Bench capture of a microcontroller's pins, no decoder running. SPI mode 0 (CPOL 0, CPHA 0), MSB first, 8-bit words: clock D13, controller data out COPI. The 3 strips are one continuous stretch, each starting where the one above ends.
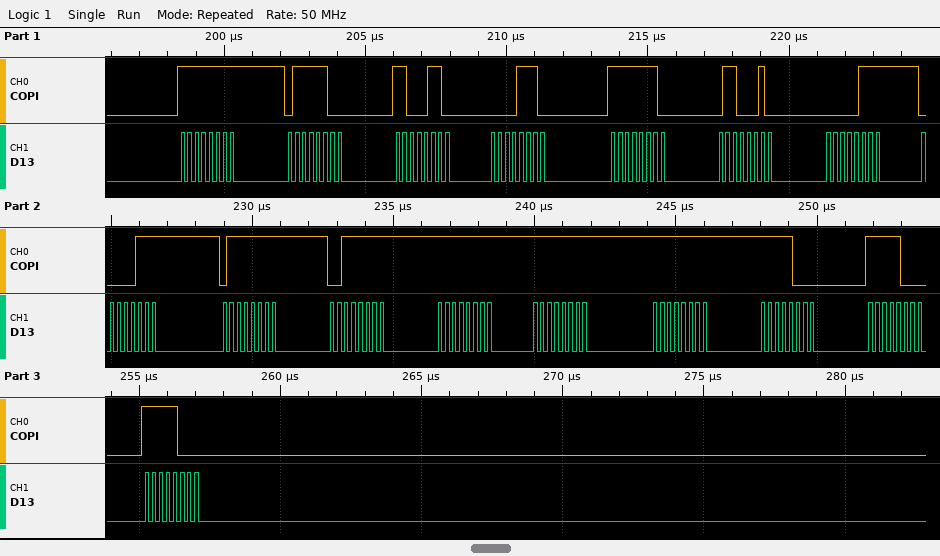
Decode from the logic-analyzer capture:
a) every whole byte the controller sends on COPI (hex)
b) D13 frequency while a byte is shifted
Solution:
0xFF 0x7C 0xC6 0x0E 0xFE 0x62 0x07 0x07 0x7F 0x3F 0xFF 0xFF 0xFF 0xF8 0xF8 0xF8
4 MHz
